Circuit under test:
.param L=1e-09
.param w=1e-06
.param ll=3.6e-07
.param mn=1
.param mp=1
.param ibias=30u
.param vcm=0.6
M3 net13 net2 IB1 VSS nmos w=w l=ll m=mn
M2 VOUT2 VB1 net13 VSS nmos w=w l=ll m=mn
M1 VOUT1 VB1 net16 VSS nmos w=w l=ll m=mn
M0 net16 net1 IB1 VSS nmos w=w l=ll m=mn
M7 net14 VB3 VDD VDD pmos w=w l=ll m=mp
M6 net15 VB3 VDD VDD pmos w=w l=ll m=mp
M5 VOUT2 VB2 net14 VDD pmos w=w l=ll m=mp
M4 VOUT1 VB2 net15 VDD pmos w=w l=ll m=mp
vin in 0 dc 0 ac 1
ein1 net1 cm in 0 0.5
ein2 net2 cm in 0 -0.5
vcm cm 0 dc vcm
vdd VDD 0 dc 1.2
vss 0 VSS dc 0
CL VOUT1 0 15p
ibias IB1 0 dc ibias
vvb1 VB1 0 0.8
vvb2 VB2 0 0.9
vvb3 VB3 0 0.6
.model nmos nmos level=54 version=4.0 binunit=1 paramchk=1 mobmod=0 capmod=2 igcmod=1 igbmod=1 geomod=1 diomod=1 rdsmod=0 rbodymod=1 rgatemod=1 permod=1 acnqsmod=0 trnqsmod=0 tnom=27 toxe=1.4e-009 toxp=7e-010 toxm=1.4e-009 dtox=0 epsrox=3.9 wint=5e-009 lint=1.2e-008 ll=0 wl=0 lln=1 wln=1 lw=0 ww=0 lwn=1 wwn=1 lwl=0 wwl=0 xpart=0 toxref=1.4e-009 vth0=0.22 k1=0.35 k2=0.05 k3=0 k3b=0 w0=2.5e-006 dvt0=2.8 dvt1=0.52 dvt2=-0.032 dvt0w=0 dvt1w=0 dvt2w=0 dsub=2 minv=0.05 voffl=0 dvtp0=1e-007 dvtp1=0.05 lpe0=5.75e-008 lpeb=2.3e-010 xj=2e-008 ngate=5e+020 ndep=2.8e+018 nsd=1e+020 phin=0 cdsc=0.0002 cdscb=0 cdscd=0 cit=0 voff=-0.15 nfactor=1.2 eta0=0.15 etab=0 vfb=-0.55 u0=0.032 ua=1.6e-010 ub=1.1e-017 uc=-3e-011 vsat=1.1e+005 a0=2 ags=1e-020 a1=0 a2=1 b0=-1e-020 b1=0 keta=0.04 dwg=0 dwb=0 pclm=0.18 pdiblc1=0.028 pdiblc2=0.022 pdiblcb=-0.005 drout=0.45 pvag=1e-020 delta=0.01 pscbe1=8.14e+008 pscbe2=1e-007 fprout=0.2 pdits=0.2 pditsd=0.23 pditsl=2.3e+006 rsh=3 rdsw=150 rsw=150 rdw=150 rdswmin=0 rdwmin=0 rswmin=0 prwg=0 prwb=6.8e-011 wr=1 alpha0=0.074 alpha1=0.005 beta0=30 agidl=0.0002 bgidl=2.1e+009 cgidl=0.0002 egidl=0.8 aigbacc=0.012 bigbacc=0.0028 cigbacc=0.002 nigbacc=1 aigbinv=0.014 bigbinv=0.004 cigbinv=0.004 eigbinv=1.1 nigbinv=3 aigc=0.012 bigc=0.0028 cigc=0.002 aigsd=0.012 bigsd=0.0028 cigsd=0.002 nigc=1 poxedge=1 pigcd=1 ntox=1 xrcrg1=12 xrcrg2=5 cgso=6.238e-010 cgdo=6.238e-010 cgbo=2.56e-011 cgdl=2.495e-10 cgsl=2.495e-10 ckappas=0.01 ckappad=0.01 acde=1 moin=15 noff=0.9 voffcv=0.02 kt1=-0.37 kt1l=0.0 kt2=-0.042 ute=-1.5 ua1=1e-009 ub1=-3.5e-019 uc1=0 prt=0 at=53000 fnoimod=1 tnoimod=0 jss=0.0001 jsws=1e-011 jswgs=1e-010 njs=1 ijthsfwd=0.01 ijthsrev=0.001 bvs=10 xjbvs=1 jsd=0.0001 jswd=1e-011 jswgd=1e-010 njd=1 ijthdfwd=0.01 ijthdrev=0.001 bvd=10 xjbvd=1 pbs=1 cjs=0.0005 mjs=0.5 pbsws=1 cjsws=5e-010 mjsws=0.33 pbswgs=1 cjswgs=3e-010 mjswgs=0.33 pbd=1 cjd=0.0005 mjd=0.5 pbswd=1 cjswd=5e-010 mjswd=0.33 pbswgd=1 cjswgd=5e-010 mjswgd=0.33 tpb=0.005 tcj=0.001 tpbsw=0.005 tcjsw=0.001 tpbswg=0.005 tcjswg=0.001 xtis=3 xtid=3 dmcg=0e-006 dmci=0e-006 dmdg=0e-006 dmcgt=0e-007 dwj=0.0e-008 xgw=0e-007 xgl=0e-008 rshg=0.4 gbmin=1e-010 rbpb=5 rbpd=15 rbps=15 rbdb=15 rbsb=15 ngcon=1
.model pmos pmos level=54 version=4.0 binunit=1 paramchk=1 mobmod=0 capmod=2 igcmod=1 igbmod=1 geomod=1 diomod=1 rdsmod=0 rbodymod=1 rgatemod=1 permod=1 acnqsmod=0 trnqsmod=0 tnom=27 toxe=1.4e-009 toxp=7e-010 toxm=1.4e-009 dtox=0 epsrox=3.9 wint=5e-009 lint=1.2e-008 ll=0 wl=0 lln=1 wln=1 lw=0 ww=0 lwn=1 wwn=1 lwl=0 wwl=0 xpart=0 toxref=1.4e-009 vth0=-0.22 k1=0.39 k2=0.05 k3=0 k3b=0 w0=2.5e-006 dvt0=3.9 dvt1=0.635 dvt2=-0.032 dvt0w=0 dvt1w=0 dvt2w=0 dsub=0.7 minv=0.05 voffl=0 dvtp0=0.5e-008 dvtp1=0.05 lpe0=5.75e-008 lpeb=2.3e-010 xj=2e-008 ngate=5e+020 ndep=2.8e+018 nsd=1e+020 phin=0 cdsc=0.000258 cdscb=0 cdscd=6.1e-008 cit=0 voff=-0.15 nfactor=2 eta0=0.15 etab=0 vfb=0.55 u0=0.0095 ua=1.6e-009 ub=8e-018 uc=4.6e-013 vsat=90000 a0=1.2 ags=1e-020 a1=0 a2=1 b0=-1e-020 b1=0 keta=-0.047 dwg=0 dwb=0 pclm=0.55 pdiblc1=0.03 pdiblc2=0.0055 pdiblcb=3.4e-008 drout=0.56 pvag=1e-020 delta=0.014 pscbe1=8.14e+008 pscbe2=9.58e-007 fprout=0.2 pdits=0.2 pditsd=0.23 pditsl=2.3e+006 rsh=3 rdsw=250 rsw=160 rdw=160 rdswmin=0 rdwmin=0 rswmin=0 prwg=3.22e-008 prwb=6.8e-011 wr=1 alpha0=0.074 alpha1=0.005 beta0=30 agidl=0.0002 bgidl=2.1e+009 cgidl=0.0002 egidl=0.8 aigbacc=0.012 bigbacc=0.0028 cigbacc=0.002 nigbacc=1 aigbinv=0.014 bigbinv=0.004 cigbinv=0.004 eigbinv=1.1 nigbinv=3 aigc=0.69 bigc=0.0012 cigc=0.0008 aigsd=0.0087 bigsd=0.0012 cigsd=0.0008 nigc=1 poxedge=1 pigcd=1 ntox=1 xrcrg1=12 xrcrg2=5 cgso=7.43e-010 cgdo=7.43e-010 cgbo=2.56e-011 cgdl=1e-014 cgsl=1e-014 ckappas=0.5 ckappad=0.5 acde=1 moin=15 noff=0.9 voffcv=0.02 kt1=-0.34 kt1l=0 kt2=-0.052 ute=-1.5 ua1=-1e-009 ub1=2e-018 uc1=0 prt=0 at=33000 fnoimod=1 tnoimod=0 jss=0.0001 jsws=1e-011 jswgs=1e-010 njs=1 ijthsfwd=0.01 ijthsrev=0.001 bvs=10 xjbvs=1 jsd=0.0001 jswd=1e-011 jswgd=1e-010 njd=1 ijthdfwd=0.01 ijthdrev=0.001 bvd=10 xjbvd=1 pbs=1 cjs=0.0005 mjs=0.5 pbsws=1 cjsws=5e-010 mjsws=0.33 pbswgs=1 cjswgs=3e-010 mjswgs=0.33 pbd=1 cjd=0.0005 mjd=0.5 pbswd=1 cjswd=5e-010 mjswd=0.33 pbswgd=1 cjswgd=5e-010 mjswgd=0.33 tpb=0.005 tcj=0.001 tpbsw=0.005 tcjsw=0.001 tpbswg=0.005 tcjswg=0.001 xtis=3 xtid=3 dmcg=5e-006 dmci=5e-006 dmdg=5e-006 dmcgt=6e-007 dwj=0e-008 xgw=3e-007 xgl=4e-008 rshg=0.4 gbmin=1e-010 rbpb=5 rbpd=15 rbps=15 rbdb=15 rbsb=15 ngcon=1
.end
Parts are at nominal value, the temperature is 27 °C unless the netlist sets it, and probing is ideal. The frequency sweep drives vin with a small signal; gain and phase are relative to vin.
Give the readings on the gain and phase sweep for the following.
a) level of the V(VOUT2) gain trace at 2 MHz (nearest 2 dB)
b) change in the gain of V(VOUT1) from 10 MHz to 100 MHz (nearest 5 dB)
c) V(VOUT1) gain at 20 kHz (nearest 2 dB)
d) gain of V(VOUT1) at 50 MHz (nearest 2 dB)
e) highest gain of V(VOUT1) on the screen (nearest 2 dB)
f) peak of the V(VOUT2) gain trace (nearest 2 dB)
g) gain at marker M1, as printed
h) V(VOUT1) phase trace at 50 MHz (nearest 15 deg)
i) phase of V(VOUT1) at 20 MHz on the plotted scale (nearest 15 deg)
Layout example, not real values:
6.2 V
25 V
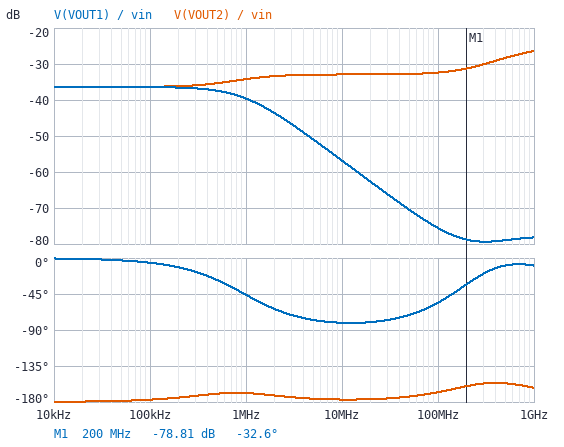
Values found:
-34 dB
-20 dB
-36 dB
-70 dB
-36 dB
-26 dB
-78.81 dB
-75 deg
-75 deg
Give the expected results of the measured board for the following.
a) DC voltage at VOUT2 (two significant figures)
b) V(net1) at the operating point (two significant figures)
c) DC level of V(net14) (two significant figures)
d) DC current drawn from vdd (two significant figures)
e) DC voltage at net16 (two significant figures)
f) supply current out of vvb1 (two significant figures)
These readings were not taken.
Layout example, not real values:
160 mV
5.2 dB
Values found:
-300 mV
600 mV
1.2 V
1.9 µA
-320 mV
19 µA
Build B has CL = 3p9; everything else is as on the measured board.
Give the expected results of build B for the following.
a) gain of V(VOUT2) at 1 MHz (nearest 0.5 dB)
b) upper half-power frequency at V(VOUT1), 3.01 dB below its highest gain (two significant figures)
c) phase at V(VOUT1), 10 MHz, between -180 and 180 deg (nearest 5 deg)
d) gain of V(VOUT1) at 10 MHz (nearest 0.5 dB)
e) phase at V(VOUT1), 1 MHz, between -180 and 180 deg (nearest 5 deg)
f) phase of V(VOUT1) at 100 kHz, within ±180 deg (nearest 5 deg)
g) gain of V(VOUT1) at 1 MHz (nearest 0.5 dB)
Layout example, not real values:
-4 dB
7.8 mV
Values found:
-36.0 dB
3.6 MHz
-65 deg
-45.5 dB
-15 deg
0 deg
-36.5 dB
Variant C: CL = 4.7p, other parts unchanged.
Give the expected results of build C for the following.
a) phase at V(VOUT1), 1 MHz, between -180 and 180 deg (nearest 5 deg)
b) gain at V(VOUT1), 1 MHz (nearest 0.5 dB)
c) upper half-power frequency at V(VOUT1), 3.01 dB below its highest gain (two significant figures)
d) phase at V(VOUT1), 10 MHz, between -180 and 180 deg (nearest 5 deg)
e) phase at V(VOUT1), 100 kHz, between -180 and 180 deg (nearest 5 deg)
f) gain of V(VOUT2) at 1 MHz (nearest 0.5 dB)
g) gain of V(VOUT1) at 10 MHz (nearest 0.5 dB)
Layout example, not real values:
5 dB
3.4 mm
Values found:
-20 deg
-37.0 dB
3.0 MHz
-70 deg
0 deg
-36.0 dB
-47.0 dB
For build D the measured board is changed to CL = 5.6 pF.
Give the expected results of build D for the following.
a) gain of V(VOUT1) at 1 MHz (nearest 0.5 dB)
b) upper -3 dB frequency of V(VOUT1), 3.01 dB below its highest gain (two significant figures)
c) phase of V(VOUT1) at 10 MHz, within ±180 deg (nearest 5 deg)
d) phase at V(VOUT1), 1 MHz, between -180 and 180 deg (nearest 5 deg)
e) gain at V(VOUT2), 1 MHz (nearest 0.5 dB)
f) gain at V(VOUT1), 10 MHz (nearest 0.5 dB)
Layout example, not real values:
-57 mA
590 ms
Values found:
-37.0 dB
2.5 MHz
-70 deg
-20 deg
-35.5 dB
-48.5 dB
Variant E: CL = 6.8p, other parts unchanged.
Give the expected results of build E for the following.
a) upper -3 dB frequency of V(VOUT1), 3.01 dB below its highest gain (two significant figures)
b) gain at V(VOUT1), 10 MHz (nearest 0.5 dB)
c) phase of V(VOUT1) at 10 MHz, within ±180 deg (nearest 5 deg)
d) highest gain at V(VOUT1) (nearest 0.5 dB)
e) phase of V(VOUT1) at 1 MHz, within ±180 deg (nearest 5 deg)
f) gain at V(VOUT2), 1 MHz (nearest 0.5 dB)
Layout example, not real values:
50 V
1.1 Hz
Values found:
2.1 MHz
-50.0 dB
-75 deg
-36.5 dB
-25 deg
-35.5 dB
